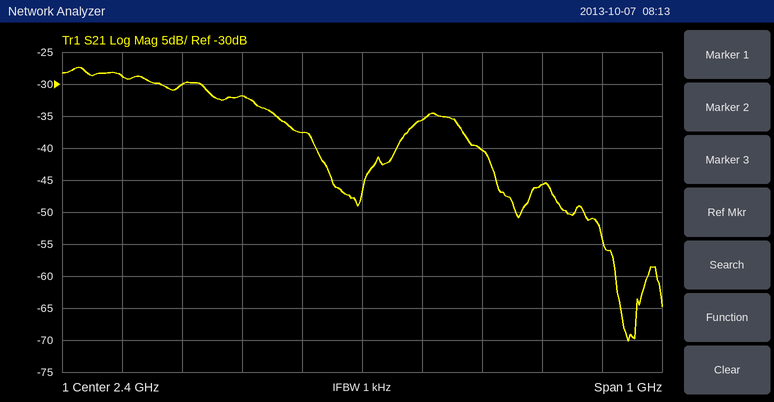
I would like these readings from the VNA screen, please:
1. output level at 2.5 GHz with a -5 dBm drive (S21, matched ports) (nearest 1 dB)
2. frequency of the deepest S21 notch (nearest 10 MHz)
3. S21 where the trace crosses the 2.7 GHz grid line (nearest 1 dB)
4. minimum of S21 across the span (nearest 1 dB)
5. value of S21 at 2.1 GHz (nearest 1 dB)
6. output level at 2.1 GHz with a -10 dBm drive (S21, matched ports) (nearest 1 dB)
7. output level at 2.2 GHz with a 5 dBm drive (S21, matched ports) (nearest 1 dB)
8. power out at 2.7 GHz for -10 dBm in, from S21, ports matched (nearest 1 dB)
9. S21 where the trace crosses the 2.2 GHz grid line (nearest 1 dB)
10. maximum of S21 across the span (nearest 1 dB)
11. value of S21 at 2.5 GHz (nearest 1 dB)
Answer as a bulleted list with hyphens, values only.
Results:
- -41 dBm
- 2.84 GHz
- -46 dB
- -70 dB
- -30 dB
- -40 dBm
- -27 dBm
- -56 dBm
- -32 dB
- -27 dB
- -36 dB
